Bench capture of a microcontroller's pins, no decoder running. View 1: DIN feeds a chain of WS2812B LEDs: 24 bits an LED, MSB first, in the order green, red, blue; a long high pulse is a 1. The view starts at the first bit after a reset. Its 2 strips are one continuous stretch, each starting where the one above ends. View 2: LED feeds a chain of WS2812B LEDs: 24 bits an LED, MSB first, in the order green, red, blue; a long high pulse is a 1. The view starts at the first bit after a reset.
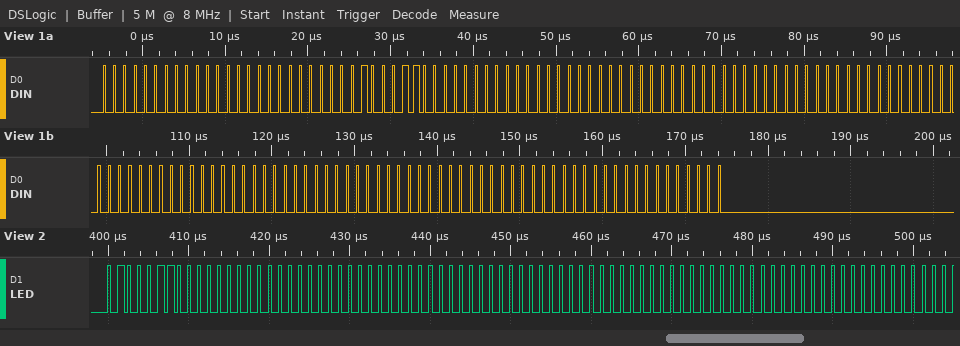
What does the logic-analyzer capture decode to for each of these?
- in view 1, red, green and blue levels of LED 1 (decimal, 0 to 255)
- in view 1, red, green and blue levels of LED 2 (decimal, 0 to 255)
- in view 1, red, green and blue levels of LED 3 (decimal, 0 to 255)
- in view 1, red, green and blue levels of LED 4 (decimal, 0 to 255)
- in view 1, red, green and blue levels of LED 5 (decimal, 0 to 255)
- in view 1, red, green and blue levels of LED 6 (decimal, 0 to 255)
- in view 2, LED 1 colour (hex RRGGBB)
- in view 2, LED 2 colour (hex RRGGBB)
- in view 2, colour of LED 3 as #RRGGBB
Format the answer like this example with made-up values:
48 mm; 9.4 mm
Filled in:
0, 0, 0; 0, 70, 0; 0, 0, 0; 0, 0, 0; 0, 0, 0; 0, 0, 0; #004600; #000000; #000000
